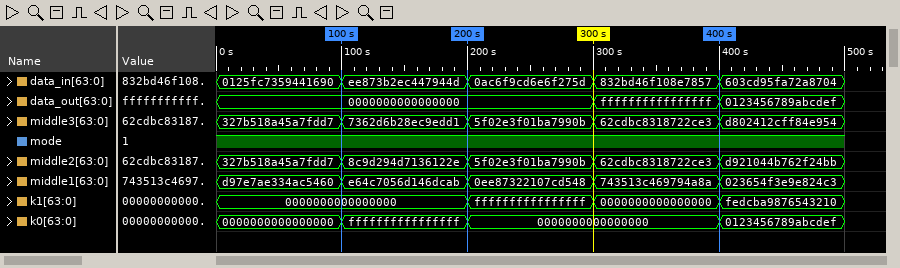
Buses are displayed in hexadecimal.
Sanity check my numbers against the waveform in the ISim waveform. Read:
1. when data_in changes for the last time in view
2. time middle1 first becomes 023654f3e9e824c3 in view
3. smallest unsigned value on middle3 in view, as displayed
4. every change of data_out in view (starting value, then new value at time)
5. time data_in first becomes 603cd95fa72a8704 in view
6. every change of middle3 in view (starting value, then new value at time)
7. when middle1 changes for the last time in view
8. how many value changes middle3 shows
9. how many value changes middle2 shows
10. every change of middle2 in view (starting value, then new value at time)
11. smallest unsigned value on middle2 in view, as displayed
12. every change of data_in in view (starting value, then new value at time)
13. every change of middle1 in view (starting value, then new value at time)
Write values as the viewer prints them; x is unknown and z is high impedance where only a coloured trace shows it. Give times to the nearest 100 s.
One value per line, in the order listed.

400 s
400 s
327b518a45a7fdd7
0000000000000000, ffffffffffffffff at 300 s, 0123456789abcdef at 400 s
400 s
327b518a45a7fdd7, 7362d6b28ec9edd1 at 100 s, 5f02e3f01ba7990b at 200 s, 62cdbc8318722ce3 at 300 s, d802412cff84e954 at 400 s
400 s
4
4
327b518a45a7fdd7, 8c9d294d7136122e at 100 s, 5f02e3f01ba7990b at 200 s, 62cdbc8318722ce3 at 300 s, d921044b762f24bb at 400 s
327b518a45a7fdd7
0125fc7359441690, ee873b2ec447944d at 100 s, 0ac6f9cd6e6f275d at 200 s, 832bd46f108e7857 at 300 s, 603cd95fa72a8704 at 400 s
d97e7ae334ac5460, e64c7056d146dcab at 100 s, 0ee87322107cd548 at 200 s, 743513c469794a8a at 300 s, 023654f3e9e824c3 at 400 s
